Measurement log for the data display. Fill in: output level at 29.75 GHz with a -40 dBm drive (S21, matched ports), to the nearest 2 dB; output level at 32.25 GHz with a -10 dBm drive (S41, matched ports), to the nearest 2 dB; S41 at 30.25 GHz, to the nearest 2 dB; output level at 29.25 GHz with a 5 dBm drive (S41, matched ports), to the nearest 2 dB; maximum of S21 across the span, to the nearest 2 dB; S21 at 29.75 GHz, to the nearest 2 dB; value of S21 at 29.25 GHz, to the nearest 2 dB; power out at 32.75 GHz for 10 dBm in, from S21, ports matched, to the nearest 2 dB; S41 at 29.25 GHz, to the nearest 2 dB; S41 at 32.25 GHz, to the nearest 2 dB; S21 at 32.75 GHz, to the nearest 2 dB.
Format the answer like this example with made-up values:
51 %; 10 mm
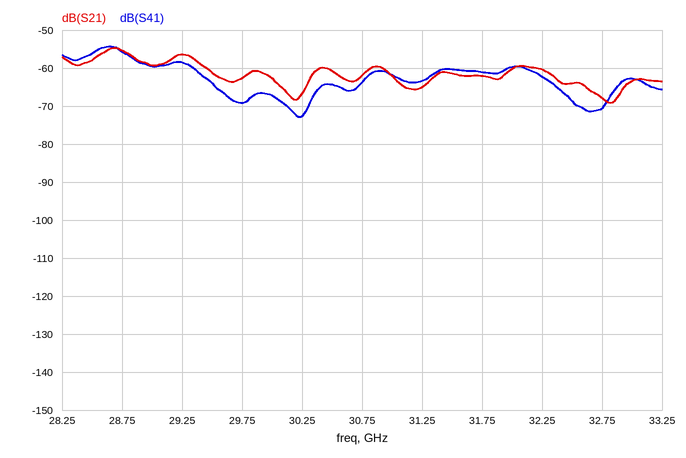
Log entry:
-102 dBm; -72 dBm; -72 dB; -54 dBm; -54 dB; -62 dB; -56 dB; -58 dBm; -58 dB; -62 dB; -68 dB
